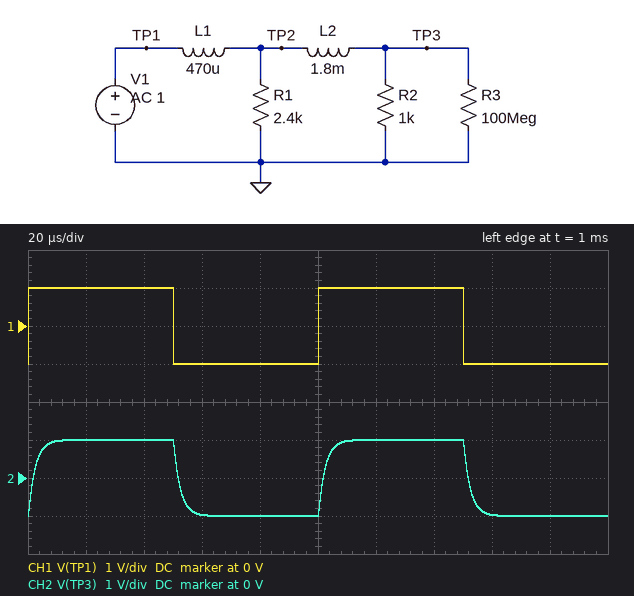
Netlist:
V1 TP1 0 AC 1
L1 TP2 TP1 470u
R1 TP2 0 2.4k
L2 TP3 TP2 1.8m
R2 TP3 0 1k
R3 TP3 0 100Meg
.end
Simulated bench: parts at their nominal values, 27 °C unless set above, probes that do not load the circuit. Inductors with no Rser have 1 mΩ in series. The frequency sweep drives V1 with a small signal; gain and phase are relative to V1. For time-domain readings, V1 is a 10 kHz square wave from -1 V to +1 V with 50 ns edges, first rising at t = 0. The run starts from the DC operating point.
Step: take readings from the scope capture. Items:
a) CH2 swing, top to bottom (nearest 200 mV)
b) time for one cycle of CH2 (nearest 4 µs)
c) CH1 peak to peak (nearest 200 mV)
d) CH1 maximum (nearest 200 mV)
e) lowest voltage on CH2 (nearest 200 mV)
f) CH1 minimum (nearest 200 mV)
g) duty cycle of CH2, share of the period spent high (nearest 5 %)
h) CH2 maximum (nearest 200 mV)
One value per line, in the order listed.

2.0 V
100 µs
2.0 V
1.0 V
-1.0 V
-1.0 V
50 %
1.0 V
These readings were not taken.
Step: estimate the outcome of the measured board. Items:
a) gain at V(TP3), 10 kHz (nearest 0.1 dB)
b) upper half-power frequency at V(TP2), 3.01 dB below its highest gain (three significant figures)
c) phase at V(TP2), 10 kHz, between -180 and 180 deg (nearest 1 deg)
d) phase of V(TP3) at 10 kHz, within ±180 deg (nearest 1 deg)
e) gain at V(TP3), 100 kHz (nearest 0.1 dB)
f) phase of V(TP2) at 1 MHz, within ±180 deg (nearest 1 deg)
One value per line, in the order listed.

-0.1 dB
496 kHz
-2 deg
-9 deg
-5.0 dB
-45 deg
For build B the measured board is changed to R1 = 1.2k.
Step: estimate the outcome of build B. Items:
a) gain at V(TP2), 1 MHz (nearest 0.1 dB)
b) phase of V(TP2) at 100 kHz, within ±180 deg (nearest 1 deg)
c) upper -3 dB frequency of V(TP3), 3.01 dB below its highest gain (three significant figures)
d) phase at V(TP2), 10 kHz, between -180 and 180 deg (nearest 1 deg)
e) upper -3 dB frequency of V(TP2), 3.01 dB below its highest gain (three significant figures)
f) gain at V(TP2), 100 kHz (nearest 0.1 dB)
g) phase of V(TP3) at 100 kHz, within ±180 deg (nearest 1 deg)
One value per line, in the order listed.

-8.9 dB
-18 deg
66.3 kHz
-3 deg
249 kHz
-1.6 dB
-67 deg
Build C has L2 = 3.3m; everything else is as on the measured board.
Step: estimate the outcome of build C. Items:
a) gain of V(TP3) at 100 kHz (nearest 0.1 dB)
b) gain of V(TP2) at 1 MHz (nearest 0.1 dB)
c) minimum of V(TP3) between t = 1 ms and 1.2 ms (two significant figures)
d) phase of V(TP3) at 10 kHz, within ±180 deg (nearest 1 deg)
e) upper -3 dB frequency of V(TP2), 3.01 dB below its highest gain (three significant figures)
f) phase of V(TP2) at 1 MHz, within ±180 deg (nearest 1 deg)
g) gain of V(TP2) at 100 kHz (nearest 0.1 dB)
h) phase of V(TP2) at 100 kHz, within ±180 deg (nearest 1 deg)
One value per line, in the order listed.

-8.3 dB
-4.5 dB
-1.0 V
-14 deg
670 kHz
-47 deg
-1.1 dB
-9 deg
